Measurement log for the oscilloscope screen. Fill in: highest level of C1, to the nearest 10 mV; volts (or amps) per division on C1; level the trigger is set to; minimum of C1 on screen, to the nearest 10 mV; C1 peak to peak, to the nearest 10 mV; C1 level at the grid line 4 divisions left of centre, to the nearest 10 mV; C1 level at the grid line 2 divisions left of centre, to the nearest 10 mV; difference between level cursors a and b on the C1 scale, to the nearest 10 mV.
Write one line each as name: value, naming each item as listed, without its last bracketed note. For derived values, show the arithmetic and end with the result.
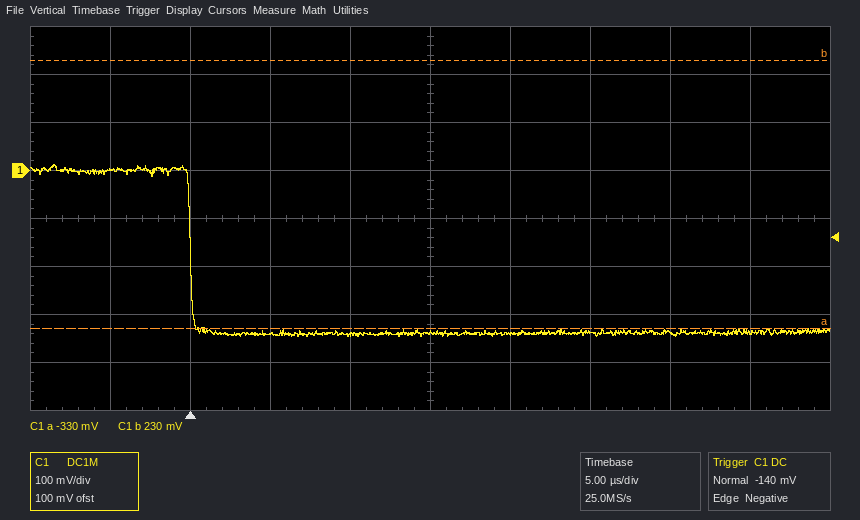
highest level of C1, to the nearest 10 mV: 10 mV
volts (or amps) per division on C1: 100 mV
level the trigger is set to: -140 mV
minimum of C1 on screen, to the nearest 10 mV: -350 mV
C1 peak to peak, to the nearest 10 mV: 10 mV − (-350 mV) = 360 mV
C1 level at the grid line 4 divisions left of centre, to the nearest 10 mV: 0 mV
C1 level at the grid line 2 divisions left of centre, to the nearest 10 mV: -340 mV
difference between level cursors a and b on the C1 scale, to the nearest 10 mV: 560 mV
